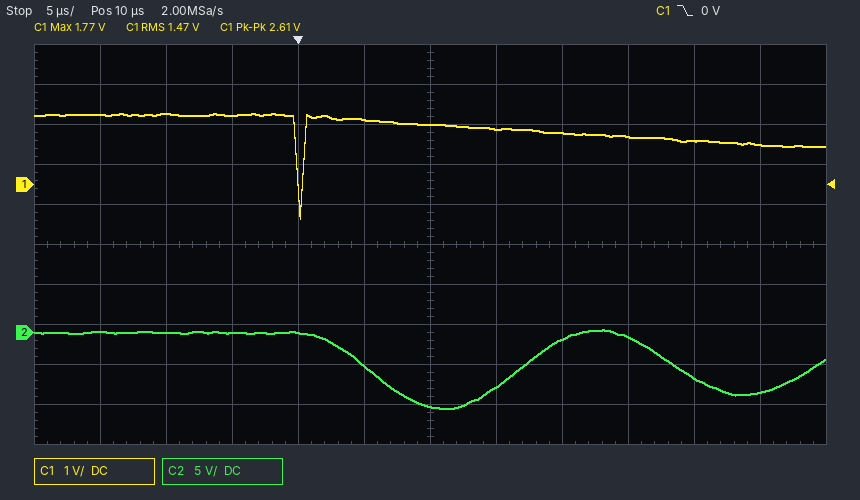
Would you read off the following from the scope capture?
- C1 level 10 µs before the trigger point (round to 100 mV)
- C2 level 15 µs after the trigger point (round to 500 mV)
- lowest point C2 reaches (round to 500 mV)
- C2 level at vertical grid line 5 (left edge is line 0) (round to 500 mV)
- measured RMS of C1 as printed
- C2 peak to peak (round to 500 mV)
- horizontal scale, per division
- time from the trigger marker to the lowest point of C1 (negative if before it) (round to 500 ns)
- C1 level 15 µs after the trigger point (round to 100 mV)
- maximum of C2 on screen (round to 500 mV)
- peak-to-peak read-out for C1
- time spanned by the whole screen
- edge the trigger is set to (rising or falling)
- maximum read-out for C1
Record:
1.8 V
-7.0 V
-9.5 V
-4.0 V
1.47 V
10.0 V
5 µs
0.0 µs
1.4 V
500 mV
2.61 V
60 µs
falling
1.77 V
